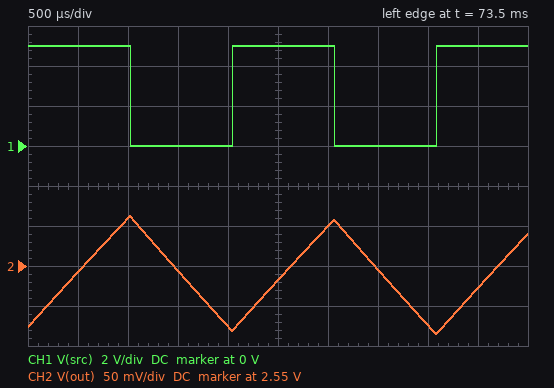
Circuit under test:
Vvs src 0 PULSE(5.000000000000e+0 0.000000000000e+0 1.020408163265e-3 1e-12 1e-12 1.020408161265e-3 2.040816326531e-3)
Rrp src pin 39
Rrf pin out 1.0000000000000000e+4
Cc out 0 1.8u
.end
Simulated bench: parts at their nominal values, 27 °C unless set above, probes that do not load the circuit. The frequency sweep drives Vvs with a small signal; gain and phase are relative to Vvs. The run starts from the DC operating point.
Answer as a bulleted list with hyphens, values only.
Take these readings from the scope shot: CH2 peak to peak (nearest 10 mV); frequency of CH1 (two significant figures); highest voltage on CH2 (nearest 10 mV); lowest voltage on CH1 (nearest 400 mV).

- 150 mV
- 490 Hz
- 2.61 V
- 0 V
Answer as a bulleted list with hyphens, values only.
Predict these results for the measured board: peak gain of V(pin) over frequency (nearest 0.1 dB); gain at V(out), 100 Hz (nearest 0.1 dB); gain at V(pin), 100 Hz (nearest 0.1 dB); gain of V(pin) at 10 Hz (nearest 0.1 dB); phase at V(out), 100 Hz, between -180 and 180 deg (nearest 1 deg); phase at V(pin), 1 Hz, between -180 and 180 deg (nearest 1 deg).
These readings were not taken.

- 0 dB
- -21.1 dB
- 0 dB
- 0 dB
- -85 deg
- 0 deg
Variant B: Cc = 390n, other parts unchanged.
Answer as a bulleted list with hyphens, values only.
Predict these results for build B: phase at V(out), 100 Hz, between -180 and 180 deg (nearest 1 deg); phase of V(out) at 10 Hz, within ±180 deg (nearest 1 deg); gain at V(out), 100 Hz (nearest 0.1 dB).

- -68 deg
- -14 deg
- -8.5 dB
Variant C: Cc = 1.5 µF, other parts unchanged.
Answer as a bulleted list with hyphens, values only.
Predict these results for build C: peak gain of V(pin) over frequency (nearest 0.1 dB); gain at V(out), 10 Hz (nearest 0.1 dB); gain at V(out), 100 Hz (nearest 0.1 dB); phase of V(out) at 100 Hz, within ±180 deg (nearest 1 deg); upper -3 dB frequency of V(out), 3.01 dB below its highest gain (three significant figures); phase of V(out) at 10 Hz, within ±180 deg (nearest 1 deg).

- 0 dB
- -2.8 dB
- -19.6 dB
- -84 deg
- 10.6 Hz
- -43 deg
